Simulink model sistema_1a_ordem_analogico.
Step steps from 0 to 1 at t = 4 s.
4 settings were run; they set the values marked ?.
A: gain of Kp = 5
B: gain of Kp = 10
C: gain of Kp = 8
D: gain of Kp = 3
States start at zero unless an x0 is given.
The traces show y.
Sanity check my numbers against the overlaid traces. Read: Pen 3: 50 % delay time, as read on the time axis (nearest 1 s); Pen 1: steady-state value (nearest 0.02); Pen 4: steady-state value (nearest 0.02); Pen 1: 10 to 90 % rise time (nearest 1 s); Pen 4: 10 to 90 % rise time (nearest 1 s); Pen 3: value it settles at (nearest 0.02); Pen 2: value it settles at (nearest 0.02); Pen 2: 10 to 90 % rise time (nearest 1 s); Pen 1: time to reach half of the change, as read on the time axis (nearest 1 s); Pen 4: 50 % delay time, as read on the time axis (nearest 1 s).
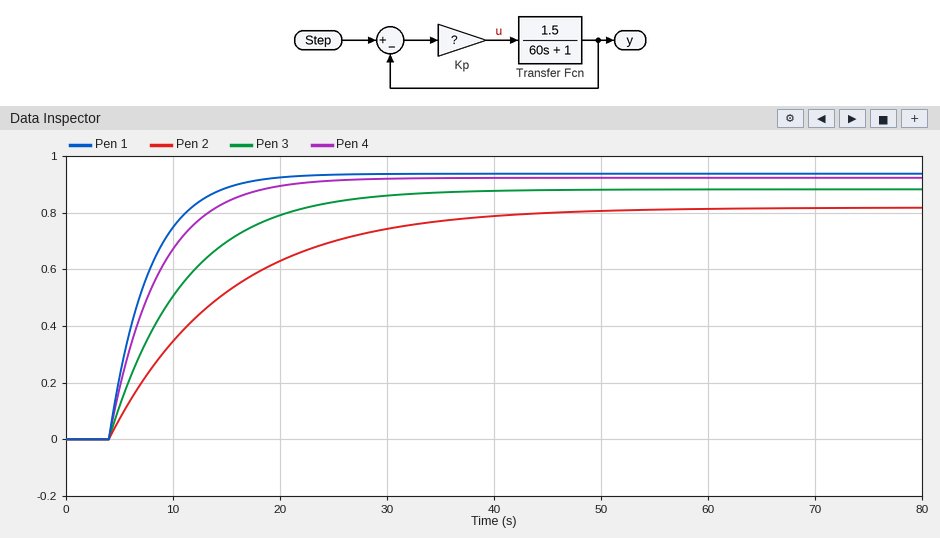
9 s
0.94
0.92
8 s
10 s
0.88
0.82
24 s
7 s
7 s
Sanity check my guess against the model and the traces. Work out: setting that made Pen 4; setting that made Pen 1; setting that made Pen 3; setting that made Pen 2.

C
B
A
D
